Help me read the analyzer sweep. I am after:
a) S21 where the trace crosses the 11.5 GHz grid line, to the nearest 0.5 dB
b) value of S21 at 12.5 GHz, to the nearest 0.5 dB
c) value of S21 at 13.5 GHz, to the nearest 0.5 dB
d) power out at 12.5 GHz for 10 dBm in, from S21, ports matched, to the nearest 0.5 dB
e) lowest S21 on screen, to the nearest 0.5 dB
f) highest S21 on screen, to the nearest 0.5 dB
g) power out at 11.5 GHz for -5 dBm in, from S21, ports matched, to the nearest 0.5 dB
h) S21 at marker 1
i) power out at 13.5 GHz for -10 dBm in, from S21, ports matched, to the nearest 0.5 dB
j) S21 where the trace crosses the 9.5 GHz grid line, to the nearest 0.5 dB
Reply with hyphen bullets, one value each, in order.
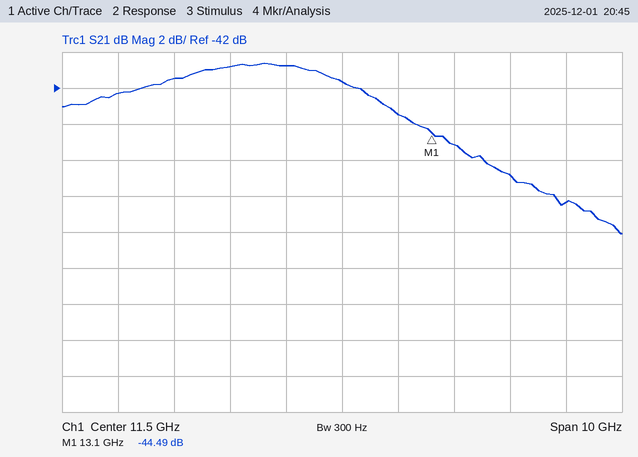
- -41.5 dB
- -43.5 dB
- -45.0 dB
- -33.5 dBm
- -50.0 dB
- -40.5 dB
- -46.5 dBm
- -44.49 dB
- -55.0 dBm
- -41.0 dB
